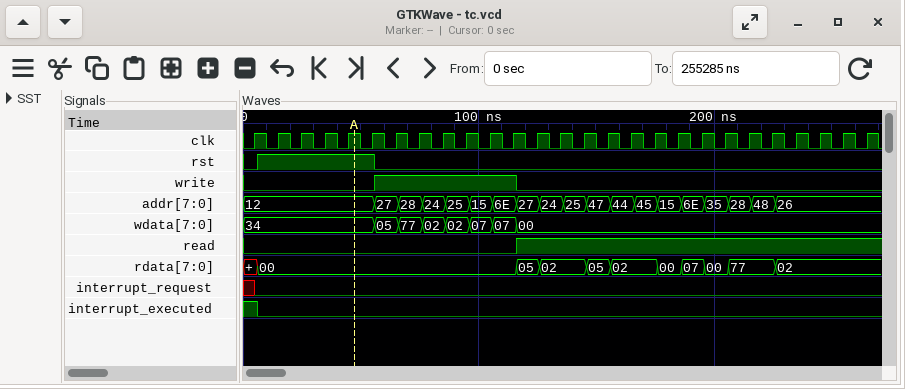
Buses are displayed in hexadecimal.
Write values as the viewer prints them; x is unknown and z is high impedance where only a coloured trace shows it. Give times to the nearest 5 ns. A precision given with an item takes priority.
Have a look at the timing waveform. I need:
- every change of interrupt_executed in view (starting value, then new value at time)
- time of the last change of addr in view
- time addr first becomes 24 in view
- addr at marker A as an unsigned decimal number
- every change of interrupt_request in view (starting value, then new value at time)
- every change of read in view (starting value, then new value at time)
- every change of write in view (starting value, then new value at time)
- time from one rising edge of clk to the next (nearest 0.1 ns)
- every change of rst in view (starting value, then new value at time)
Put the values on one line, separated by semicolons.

1, 0 at 5 ns; 225 ns; 75 ns; 18; x, 0 at 5 ns; 0, 1 at 115 ns; 0, 1 at 55 ns, 0 at 115 ns; 10 ns; 0, 1 at 5 ns, 0 at 55 ns
